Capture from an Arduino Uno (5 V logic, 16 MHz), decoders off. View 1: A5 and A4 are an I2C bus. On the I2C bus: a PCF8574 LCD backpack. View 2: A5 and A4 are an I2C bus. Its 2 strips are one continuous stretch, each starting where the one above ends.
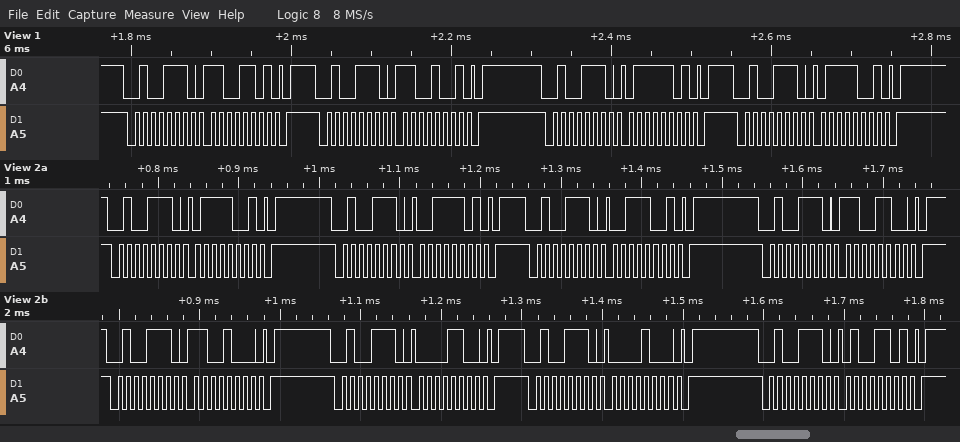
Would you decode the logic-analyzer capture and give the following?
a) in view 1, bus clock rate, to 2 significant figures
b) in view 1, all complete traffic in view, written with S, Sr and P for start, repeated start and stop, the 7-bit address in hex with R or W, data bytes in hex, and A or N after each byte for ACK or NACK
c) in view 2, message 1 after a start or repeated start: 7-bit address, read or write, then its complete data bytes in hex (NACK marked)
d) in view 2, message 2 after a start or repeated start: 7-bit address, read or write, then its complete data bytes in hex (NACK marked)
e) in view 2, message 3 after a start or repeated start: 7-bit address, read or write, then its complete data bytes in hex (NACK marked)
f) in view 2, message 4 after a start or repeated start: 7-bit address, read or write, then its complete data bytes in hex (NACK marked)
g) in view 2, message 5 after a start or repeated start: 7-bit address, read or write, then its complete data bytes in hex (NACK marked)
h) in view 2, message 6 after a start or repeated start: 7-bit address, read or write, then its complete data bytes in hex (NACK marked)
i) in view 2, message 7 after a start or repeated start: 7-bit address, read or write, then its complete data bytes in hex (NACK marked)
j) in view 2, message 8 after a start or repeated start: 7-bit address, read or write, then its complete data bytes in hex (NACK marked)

100 kHz
S 27W A CD A P S 27W A C9 A P S 27W A 7D A P S 27W A 79 A P
0x27 write: 79
0x27 write: 3D
0x27 write: 39
0x27 write: CC
0x27 write: C8
0x27 write: 0C
0x27 write: 08
0x27 write: 4D
